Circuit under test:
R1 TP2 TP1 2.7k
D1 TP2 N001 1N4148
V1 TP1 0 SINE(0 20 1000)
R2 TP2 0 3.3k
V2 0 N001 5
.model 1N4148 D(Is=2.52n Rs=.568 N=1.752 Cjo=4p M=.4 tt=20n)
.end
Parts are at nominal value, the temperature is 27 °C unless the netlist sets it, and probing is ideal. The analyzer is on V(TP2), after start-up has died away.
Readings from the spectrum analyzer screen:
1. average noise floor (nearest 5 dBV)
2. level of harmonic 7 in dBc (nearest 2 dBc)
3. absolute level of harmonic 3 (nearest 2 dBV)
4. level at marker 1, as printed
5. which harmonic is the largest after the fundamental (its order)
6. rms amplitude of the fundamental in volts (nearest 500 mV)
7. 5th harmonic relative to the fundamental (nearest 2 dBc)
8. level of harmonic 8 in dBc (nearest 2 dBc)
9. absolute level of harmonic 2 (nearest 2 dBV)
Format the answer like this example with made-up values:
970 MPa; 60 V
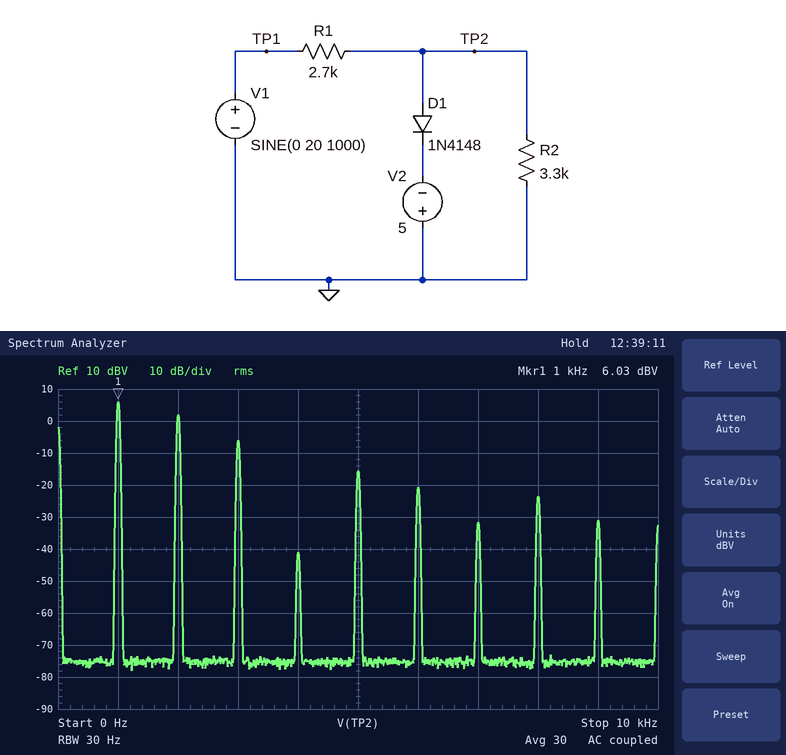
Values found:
-75 dBV; -38 dBc; -6 dBV; 6.03 dBV; 2; 2.0 V; -22 dBc; -30 dBc; 2 dBV
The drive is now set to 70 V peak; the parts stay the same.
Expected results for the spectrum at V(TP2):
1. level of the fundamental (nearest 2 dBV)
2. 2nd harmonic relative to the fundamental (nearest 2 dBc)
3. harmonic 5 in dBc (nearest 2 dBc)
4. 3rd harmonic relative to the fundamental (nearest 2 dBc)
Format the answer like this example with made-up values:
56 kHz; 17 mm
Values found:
22 dBV; -6 dBc; -30 dBc; -26 dBc
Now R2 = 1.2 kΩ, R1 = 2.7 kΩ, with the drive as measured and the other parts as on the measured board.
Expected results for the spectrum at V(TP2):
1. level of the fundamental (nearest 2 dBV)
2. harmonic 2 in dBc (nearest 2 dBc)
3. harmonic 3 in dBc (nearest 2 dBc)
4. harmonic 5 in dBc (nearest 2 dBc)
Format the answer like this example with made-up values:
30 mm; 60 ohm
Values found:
-8 dBV; -2 dBc; -6 dBc; -20 dBc
